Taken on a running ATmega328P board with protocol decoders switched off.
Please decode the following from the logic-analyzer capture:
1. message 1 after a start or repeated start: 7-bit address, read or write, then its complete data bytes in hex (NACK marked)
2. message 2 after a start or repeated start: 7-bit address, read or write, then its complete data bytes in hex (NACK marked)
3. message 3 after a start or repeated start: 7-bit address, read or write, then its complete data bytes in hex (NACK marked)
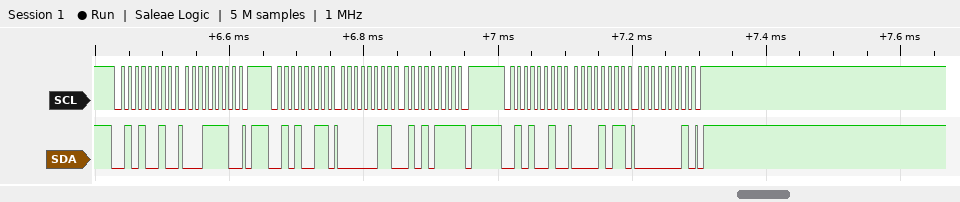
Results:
0x29 write: 1E
0x29 read: 03 57 NACK
0x29 write: 0B 01
